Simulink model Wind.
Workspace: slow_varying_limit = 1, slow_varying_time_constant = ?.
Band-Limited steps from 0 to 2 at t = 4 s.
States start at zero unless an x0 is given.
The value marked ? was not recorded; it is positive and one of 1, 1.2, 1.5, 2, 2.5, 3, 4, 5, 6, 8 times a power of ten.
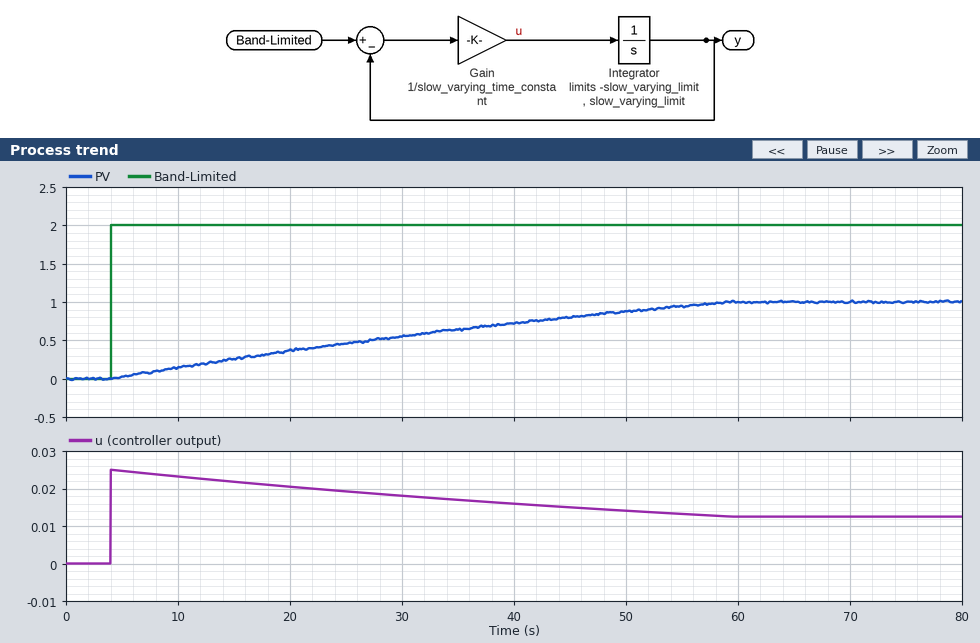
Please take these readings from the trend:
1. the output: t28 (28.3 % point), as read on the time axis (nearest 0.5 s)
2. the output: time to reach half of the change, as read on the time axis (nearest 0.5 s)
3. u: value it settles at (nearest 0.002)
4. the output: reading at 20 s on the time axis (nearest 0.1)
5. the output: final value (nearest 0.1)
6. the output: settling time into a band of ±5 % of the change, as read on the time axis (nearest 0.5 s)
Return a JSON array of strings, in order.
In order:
["16.0 s", "27.0 s", "0.012", "0.4", "1.0", "55.5 s"]
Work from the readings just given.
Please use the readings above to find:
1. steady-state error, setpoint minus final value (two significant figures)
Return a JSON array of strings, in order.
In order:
["1.0"]
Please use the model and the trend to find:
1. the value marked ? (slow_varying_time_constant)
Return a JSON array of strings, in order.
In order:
["80"]
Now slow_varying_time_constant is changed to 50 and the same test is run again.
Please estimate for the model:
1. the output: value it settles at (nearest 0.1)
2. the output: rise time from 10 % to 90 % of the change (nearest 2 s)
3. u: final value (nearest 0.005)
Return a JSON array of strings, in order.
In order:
["1.0", "28 s", "0.020"]
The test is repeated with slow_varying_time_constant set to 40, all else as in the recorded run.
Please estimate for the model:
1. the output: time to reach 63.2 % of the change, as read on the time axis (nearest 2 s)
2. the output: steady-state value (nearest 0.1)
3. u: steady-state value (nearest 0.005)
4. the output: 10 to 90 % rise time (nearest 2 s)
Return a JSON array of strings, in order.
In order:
["20 s", "1.0", "0.025", "22 s"]
